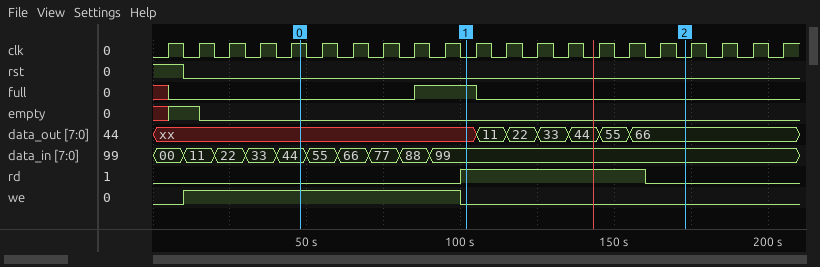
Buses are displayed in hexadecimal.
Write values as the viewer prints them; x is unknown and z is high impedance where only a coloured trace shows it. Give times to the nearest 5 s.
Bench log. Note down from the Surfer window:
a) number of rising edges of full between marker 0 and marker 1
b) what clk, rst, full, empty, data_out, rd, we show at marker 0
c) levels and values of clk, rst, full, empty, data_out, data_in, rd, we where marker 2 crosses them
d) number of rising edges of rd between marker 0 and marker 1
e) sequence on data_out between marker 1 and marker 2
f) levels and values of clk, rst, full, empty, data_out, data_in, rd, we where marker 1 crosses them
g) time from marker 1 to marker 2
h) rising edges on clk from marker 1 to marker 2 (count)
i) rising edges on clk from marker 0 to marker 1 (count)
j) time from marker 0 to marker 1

1
clk=1, rst=0, full=0, empty=0, data_out=xx, rd=0, we=1
clk=0, rst=0, full=0, empty=0, data_out=66, data_in=99, rd=0, we=0
1
xx, 11, 22, 33, 44, 55, 66
clk=0, rst=0, full=1, empty=0, data_out=xx, data_in=99, rd=1, we=0
70 s
7
5
55 s
